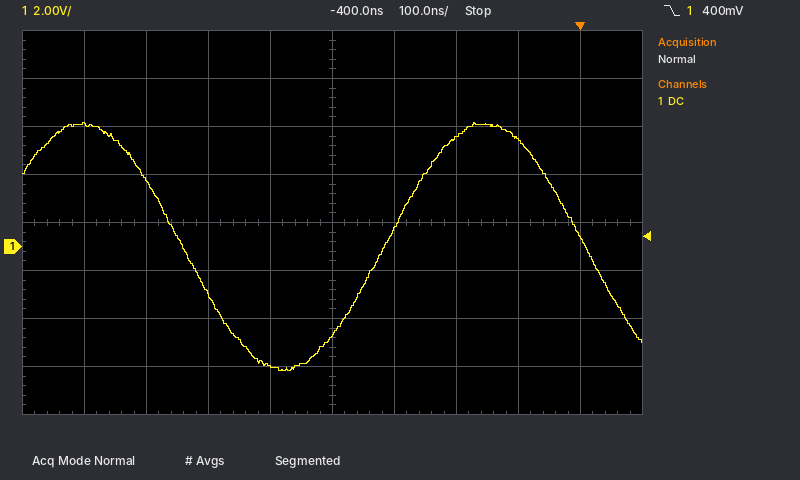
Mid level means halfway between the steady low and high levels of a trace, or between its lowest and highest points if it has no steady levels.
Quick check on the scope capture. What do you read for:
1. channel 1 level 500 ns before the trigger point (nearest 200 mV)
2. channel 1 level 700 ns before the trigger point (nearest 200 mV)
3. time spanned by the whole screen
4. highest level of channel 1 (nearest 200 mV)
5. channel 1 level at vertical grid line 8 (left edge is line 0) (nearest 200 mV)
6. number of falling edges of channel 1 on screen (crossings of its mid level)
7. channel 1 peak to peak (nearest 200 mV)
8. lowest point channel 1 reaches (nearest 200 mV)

-5.0 V
2.8 V
1 µs
5.2 V
4.4 V
2
10.4 V
-5.2 V
